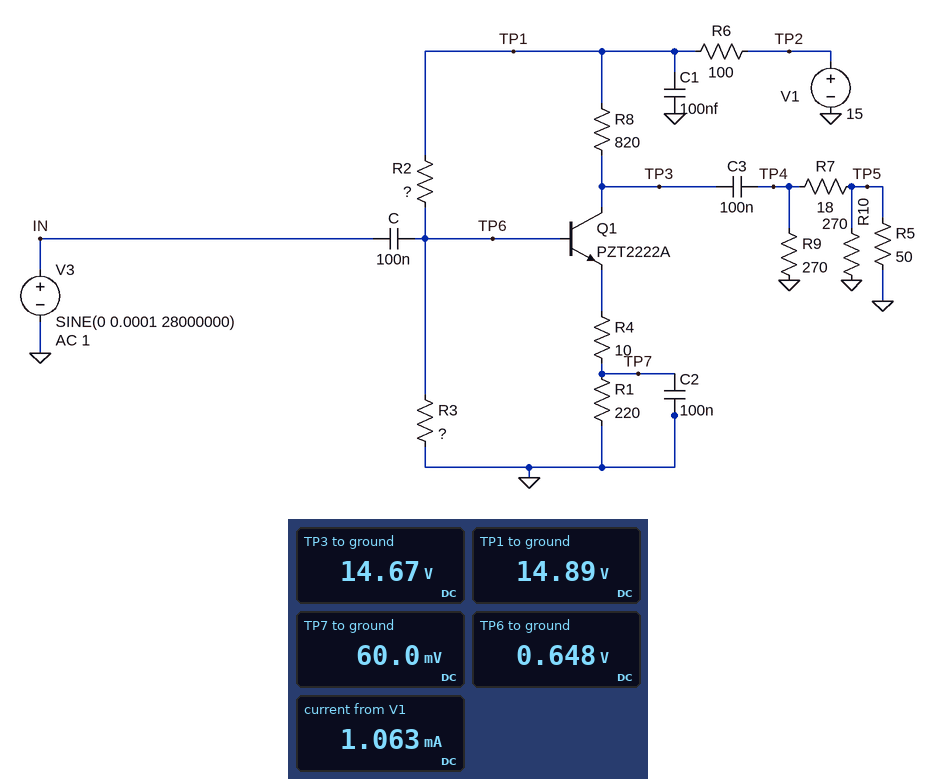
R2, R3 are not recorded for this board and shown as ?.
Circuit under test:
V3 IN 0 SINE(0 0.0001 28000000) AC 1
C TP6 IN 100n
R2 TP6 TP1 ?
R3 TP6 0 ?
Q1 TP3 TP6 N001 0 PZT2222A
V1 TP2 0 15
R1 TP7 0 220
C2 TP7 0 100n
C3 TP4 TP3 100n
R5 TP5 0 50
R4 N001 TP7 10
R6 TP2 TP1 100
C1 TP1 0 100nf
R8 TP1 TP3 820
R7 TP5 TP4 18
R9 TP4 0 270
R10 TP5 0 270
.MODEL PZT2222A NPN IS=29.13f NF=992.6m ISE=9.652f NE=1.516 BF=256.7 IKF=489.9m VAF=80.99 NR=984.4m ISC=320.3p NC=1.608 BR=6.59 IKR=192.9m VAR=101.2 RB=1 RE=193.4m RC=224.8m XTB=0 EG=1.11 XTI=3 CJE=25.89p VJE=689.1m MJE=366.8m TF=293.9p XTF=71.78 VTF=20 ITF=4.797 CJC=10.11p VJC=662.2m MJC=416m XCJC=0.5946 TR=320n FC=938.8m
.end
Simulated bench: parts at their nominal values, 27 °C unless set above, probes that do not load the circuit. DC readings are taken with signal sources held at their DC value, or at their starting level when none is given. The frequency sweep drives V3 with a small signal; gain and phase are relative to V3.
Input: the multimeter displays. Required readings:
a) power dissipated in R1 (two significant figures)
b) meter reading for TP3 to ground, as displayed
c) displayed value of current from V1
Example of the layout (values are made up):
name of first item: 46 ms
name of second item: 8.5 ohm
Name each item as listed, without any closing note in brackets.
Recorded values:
power dissipated in R1: 16 µW
meter reading for TP3 to ground, as displayed: 14.67 V
displayed value of current from V1: 1.063 mA
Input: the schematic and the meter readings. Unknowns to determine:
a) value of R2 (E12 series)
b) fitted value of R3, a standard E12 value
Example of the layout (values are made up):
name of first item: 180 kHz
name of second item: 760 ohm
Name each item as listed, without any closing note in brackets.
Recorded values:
value of R2: 18 kΩ
fitted value of R3, a standard E12 value: 820 Ω
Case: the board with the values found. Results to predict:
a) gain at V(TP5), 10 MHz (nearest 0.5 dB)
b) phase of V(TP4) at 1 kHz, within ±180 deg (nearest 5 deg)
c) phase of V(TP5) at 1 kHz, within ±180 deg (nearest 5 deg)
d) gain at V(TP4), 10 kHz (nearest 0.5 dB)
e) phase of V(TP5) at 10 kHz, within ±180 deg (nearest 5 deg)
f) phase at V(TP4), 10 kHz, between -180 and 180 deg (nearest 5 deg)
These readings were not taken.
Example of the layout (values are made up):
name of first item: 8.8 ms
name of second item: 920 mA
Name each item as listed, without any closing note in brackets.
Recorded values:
gain at V(TP5), 10 MHz: -10.0 dB
phase of V(TP4) at 1 kHz, within ±180 deg: -50 deg
phase of V(TP5) at 1 kHz, within ±180 deg: -50 deg
gain at V(TP4), 10 kHz: -13.5 dB
phase of V(TP5) at 10 kHz, within ±180 deg: -130 deg
phase at V(TP4), 10 kHz, between -180 and 180 deg: -130 deg
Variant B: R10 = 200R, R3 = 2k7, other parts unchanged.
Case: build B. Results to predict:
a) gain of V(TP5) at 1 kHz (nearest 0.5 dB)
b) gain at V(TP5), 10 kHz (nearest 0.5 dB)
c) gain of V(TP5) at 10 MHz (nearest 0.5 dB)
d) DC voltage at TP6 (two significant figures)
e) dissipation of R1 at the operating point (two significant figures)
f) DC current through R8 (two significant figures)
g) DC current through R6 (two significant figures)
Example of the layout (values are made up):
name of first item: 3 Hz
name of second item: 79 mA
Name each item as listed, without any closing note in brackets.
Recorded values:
gain of V(TP5) at 1 kHz: -25.0 dB
gain at V(TP5), 10 kHz: -13.0 dB
gain of V(TP5) at 10 MHz: 6.0 dB
DC voltage at TP6: 1.8 V
dissipation of R1 at the operating point: 5.7 mW
DC current through R8: 5.1 mA
DC current through R6: 5.8 mA
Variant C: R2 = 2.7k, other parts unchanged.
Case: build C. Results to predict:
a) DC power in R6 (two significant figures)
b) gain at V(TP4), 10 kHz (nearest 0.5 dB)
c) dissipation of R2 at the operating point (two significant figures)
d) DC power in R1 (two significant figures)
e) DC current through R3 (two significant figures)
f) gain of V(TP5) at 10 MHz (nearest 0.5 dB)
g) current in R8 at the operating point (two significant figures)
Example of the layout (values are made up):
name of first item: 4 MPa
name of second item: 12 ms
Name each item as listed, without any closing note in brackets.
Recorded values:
DC power in R6: 21 mW
gain at V(TP4), 10 kHz: -10.0 dB
dissipation of R2 at the operating point: 40 mW
DC power in R1: 25 mW
DC current through R3: 3.8 mA
gain of V(TP5) at 10 MHz: 8.0 dB
current in R8 at the operating point: 11 mA
